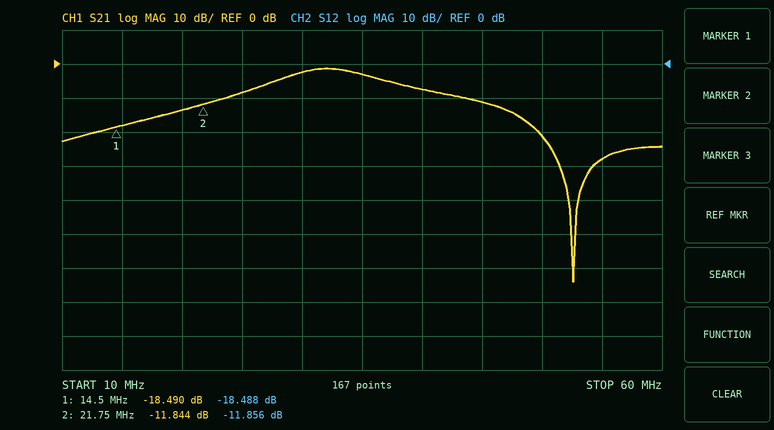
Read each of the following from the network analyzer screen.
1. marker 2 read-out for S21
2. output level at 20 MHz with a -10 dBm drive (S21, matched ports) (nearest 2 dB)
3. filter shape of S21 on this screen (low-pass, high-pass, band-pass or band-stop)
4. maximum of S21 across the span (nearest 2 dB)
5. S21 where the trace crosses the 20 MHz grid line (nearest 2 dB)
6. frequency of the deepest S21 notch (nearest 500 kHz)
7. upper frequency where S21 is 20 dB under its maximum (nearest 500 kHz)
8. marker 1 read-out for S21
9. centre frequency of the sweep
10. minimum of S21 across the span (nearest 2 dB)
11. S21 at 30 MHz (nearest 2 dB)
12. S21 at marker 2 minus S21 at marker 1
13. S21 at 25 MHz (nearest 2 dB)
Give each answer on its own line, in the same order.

-11.844 dB
-24 dBm
band-pass
-2 dB
-14 dB
52.5 MHz
50.0 MHz
-18.490 dB
35 MHz
-64 dB
-2 dB
6.646 dB
-8 dB
